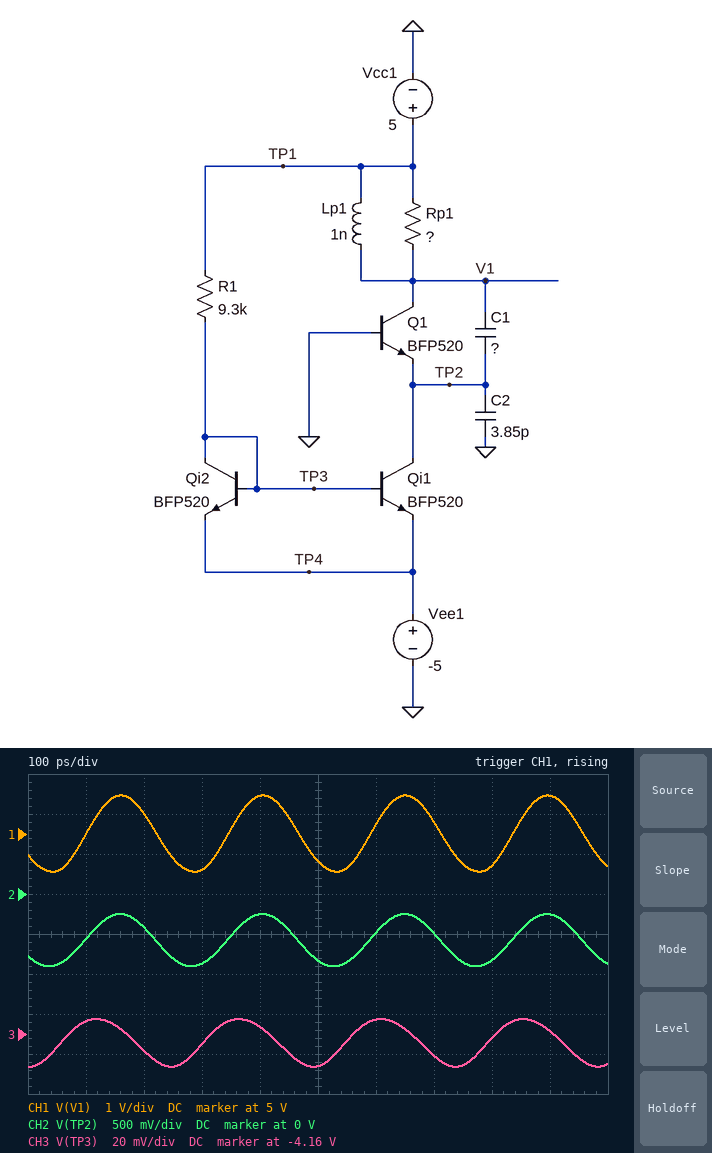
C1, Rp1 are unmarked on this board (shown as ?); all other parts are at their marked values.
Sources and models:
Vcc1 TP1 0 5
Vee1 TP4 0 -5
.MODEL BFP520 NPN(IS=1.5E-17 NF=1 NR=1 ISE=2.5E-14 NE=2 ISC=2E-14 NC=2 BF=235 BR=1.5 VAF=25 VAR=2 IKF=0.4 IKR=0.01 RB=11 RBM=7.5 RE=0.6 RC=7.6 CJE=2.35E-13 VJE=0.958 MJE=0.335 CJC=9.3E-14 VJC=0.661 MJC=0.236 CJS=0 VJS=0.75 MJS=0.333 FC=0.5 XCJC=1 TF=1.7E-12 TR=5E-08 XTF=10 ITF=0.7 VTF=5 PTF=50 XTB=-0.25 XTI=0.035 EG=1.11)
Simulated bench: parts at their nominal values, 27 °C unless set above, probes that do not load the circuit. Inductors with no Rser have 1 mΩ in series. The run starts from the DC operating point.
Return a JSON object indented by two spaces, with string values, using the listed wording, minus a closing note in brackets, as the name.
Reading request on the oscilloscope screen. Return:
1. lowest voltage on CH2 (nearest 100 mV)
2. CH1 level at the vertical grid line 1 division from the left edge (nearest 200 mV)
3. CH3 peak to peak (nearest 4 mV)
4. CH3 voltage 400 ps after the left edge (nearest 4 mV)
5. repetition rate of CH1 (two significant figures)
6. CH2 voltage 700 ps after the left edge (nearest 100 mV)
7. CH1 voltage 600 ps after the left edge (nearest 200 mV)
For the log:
{
  "lowest voltage on CH2": "-900 mV",
  "CH1 level at the vertical grid line 1 division from the left edge": "5.0 V",
  "CH3 peak to peak": "24 mV",
  "CH3 voltage 400 ps after the left edge": "-4.156 V",
  "repetition rate of CH1": "4.1 GHz",
  "CH2 voltage 700 ps after the left edge": "-500 mV",
  "CH1 voltage 600 ps after the left edge": "5.2 V"
}
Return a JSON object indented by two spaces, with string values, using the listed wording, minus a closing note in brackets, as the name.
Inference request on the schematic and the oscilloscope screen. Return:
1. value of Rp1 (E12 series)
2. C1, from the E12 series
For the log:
{
  "value of Rp1": "820 Ω",
  "C1, from the E12 series": "2.2 pF"
}
